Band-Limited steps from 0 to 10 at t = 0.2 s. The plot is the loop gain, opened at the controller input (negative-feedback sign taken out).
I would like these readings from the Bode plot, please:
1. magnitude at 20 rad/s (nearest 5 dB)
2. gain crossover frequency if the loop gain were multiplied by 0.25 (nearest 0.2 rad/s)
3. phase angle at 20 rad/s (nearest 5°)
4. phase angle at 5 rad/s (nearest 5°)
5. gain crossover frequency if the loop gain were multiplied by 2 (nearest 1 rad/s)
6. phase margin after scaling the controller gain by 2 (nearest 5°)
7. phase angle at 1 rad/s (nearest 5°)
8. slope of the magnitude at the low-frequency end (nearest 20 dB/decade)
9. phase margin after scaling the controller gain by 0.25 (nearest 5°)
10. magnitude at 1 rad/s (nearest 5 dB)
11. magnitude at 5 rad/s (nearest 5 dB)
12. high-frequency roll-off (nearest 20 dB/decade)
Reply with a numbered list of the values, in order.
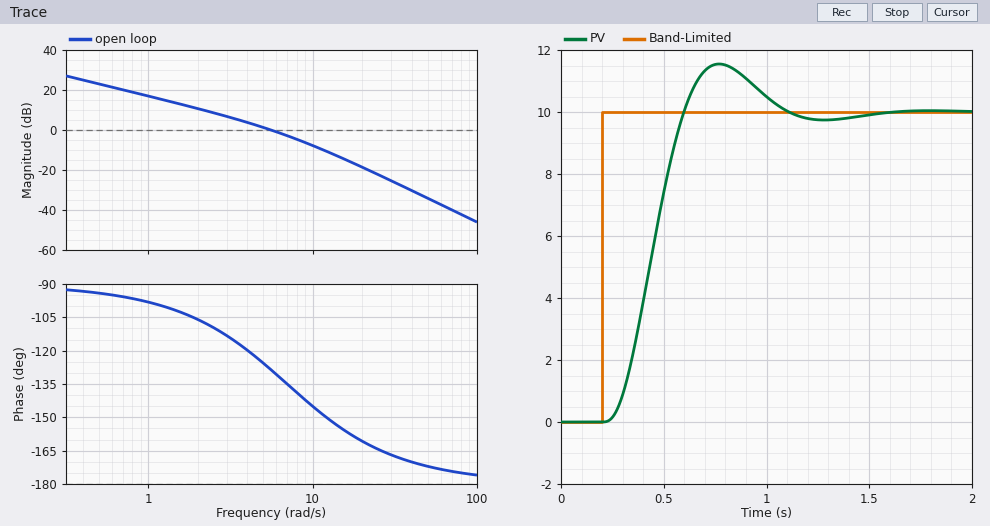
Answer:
1. -20 dB
2. 1.8 rad/s
3. -160°
4. -125°
5. 9 rad/s
6. 40°
7. -100°
8. -20 dB/decade
9. 75°
10. 15 dB
11. 0 dB
12. -40 dB/decade
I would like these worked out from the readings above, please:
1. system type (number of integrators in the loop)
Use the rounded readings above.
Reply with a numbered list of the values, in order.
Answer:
1. 1
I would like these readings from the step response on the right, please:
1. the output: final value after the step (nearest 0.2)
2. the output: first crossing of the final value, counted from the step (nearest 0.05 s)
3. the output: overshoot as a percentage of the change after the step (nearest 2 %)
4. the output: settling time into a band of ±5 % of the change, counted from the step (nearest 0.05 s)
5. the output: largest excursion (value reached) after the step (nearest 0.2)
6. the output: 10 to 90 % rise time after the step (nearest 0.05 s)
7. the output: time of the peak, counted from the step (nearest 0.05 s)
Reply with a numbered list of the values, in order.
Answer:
1. 10.0
2. 0.40 s
3. 16 %
4. 0.80 s
5. 11.6
6. 0.25 s
7. 0.55 s
